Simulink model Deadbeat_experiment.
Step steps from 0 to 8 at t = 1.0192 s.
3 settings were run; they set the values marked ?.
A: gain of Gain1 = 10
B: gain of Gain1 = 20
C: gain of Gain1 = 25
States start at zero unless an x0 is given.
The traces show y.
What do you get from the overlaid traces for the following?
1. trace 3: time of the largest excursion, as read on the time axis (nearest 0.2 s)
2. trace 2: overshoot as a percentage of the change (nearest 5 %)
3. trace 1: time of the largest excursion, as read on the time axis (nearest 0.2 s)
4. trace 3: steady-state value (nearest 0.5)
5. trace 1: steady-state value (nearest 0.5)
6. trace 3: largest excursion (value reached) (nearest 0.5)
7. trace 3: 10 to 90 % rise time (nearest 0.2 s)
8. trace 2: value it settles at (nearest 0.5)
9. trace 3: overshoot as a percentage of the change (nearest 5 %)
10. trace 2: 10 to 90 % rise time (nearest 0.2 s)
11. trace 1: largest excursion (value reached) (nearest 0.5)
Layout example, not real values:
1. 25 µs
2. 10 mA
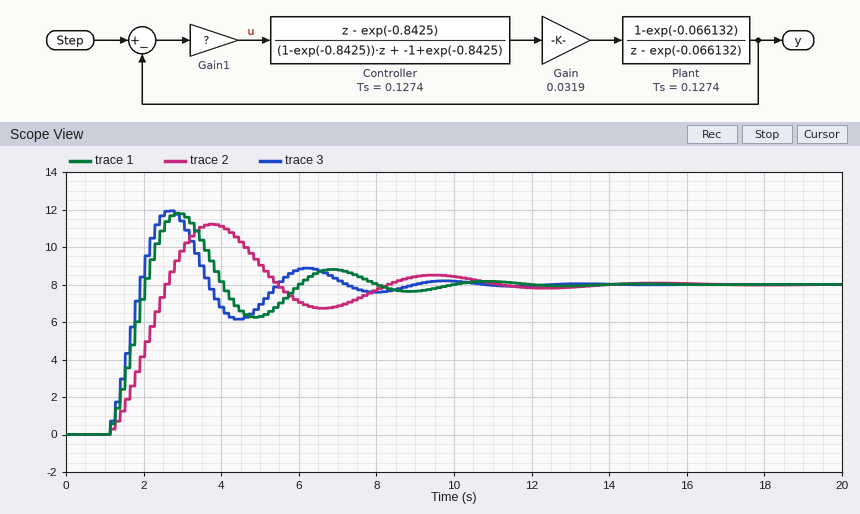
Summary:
1. 2.6 s
2. 40 %
3. 2.8 s
4. 8.0
5. 8.0
6. 12.0
7. 0.6 s
8. 8.0
9. 50 %
10. 1.0 s
11. 12.0
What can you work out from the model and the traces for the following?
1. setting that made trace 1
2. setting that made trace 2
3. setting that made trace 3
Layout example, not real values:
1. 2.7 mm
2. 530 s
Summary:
1. B
2. A
3. C
